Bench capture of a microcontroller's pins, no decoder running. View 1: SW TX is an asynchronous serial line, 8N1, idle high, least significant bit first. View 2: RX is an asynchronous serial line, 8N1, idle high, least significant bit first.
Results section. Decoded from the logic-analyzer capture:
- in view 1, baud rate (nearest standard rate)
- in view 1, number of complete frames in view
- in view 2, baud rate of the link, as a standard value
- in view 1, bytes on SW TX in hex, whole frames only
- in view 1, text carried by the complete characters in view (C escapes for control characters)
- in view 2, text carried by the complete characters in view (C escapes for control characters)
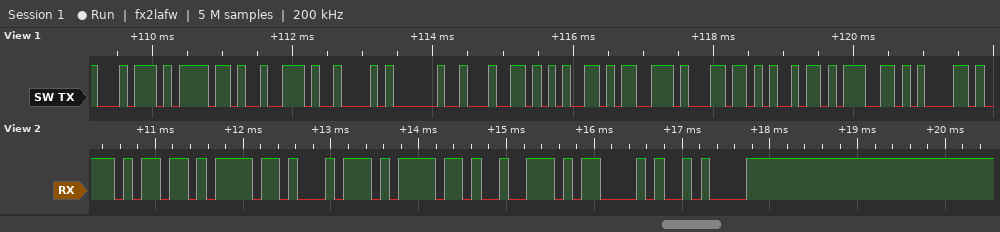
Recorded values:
9600 baud
12
9600 baud
74 6F 72 42 20 64 65 73 6C 69 67 61
"torB desliga"
"motorC\n"
